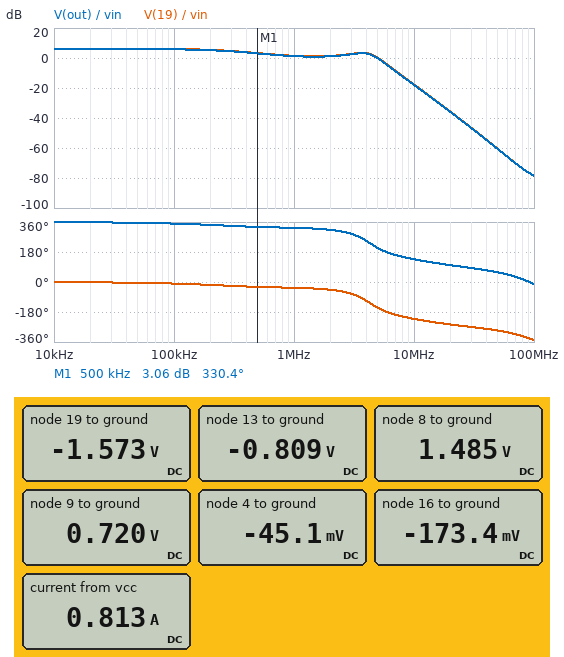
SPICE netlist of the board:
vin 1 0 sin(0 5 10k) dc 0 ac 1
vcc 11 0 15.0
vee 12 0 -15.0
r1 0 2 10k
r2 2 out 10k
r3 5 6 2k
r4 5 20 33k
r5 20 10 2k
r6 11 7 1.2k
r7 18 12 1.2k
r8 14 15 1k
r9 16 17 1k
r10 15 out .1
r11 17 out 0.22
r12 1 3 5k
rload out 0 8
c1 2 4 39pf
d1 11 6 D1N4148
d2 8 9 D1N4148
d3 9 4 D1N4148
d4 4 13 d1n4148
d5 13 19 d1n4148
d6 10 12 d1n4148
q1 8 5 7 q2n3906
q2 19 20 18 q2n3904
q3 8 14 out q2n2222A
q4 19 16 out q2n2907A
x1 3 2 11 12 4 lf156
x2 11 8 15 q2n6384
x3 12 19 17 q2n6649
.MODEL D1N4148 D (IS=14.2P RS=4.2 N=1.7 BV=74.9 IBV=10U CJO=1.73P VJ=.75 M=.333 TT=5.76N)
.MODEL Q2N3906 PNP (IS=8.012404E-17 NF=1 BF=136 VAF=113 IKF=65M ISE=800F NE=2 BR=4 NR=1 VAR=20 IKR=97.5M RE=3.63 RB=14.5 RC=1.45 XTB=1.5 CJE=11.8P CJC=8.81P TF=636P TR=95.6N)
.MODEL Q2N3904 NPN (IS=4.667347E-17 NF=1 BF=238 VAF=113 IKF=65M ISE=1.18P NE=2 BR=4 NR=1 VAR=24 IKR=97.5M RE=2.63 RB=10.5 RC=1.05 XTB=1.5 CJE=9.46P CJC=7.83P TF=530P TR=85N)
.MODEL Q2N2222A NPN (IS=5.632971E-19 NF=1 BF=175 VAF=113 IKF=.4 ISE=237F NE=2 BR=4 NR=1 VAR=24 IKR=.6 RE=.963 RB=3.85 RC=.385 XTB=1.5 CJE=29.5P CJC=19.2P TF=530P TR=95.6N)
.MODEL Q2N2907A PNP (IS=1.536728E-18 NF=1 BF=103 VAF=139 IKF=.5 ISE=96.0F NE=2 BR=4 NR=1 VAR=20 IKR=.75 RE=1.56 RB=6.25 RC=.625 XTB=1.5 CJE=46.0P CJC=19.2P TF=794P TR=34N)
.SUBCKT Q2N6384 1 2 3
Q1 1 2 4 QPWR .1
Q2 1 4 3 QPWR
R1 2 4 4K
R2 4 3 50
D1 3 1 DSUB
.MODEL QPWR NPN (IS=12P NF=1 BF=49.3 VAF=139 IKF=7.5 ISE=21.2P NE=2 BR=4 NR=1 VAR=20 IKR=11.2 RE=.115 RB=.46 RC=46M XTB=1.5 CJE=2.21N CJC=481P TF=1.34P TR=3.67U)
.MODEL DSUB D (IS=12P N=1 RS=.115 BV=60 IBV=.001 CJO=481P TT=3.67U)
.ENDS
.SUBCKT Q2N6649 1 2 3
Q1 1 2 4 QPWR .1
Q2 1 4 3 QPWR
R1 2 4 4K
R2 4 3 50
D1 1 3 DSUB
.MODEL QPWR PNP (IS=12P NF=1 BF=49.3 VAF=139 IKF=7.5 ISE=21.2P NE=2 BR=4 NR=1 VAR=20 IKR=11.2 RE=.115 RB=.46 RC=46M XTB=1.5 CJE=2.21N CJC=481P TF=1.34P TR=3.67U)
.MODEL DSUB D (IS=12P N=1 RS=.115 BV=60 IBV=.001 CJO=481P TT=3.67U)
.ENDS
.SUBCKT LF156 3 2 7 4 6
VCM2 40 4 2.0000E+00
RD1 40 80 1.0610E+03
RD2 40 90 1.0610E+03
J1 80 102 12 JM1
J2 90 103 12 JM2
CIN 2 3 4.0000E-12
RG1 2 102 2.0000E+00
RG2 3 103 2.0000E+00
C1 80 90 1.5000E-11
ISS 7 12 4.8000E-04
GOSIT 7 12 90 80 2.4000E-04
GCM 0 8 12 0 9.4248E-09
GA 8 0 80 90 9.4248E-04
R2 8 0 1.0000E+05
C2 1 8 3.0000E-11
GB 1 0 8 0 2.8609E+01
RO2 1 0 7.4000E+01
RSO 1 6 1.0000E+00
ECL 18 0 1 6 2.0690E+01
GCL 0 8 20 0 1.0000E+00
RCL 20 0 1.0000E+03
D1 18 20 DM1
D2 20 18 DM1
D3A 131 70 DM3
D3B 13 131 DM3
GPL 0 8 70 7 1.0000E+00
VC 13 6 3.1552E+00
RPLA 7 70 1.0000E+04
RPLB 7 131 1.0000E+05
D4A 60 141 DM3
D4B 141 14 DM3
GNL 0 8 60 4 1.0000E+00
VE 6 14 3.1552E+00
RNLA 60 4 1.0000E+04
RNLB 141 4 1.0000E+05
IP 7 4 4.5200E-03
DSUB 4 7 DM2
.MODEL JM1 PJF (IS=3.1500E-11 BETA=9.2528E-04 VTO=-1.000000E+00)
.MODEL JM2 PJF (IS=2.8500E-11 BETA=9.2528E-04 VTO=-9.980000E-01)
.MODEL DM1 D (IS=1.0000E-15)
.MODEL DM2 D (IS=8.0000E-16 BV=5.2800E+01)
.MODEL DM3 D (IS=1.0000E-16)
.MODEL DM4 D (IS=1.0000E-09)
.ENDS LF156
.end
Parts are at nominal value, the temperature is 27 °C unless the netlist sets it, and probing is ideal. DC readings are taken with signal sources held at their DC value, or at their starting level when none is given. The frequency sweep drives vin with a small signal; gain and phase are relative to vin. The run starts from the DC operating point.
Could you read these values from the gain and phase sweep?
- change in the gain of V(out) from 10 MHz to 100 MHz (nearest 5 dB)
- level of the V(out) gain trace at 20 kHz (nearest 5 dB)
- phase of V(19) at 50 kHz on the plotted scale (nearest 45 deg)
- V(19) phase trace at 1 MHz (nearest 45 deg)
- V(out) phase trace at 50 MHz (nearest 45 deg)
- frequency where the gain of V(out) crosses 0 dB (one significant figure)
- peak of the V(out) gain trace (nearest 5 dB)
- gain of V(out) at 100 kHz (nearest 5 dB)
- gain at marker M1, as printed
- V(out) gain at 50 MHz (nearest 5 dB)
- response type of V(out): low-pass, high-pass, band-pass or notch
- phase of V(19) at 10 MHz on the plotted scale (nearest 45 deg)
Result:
-60 dB
5 dB
0 deg
-45 deg
45 deg
5 MHz
5 dB
5 dB
3.06 dB
-60 dB
low-pass
-225 deg
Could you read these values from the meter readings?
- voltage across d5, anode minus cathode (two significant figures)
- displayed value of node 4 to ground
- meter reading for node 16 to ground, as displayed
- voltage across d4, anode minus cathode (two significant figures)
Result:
760 mV
-45.1 mV
-173.4 mV
760 mV
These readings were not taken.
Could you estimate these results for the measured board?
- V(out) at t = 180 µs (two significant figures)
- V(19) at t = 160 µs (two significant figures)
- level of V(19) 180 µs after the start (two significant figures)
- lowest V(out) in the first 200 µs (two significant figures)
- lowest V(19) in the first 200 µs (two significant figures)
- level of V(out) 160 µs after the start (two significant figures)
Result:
-9.6 V
-7.4 V
-11 V
-10 V
-12 V
-5.7 V
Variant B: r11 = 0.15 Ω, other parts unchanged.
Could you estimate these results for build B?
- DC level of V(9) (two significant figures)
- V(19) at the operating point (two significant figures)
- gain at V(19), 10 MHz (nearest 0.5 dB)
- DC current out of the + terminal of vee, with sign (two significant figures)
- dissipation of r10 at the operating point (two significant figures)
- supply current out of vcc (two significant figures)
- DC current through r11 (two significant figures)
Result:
740 mV
-1.5 V
-18.0 dB
-880 mA
76 mW
880 mA
870 mA
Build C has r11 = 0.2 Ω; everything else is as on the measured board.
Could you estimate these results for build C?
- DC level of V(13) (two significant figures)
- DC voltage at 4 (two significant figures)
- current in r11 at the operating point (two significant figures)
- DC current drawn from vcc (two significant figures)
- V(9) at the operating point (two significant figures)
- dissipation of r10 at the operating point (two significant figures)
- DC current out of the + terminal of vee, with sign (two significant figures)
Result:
-800 mV
-38 mV
820 mA
830 mA
730 mV
68 mW
-830 mA
